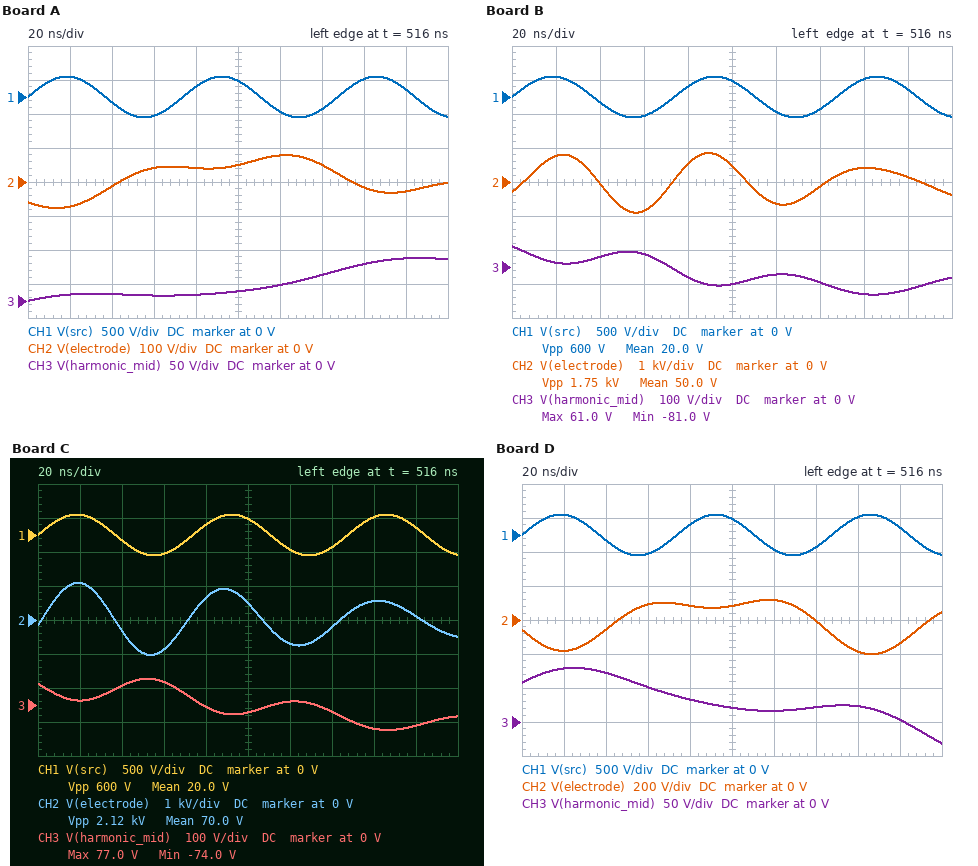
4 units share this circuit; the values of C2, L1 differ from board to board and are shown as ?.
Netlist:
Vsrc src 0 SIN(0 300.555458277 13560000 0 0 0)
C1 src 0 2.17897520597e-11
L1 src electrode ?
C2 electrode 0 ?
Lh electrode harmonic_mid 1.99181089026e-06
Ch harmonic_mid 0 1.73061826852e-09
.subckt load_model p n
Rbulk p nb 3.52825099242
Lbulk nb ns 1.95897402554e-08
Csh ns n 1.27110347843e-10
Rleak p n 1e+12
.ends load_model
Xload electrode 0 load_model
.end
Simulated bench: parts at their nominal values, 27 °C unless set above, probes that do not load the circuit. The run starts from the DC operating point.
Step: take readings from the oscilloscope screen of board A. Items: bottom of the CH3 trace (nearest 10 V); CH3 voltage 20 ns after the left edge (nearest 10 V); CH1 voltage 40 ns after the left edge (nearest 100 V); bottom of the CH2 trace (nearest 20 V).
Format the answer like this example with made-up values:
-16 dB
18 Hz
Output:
0 V
10 V
-100 V
-80 V
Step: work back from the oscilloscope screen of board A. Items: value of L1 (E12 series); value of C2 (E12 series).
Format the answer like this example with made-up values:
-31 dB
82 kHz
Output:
1.8 µH
1 nF
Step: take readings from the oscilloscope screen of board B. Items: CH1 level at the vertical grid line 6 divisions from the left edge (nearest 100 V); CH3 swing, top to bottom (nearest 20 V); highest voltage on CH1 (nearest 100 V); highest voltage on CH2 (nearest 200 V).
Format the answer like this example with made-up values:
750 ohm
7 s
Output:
-200 V
140 V
300 V
800 V
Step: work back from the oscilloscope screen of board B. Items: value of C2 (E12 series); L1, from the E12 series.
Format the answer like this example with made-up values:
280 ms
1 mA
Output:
270 pF
220 nH
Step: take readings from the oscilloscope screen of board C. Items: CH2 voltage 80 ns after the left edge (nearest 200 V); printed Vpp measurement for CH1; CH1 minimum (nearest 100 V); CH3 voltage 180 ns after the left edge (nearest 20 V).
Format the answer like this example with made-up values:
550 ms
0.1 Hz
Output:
600 V
600 V
-300 V
-60 V
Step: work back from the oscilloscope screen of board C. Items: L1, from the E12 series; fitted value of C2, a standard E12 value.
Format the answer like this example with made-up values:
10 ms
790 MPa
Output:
470 nH
120 pF
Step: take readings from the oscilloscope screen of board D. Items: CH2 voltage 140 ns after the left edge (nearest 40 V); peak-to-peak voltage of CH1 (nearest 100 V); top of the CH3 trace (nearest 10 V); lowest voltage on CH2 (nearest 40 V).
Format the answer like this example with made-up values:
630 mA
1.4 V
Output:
0 V
600 V
80 V
-200 V
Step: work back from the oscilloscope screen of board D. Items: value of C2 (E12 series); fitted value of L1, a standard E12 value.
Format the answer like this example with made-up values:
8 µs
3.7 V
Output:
820 pF
820 nH
